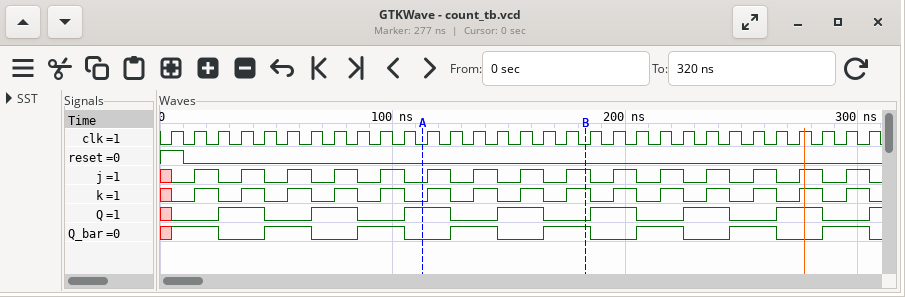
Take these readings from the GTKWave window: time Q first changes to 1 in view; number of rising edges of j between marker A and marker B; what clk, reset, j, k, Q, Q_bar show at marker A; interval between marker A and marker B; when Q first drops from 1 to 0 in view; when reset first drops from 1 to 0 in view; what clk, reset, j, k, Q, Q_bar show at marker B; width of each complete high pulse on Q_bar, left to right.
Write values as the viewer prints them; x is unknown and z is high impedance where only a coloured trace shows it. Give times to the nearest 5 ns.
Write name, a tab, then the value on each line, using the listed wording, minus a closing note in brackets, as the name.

time Q first changes to 1 in view	25 ns
number of rising edges of j between marker A and marker B	4
what clk, reset, j, k, Q, Q_bar show at marker A	clk=0, reset=0, j=0, k=0, Q=1, Q_bar=0
interval between marker A and marker B	70 ns
when Q first drops from 1 to 0 in view	45 ns
when reset first drops from 1 to 0 in view	10 ns
what clk, reset, j, k, Q, Q_bar show at marker B	clk=0, reset=0, j=1, k=1, Q=0, Q_bar=1
width of each complete high pulse on Q_bar, left to right	20 ns, 20 ns, 20 ns, 20 ns, 20 ns, 20 ns, 20 ns
